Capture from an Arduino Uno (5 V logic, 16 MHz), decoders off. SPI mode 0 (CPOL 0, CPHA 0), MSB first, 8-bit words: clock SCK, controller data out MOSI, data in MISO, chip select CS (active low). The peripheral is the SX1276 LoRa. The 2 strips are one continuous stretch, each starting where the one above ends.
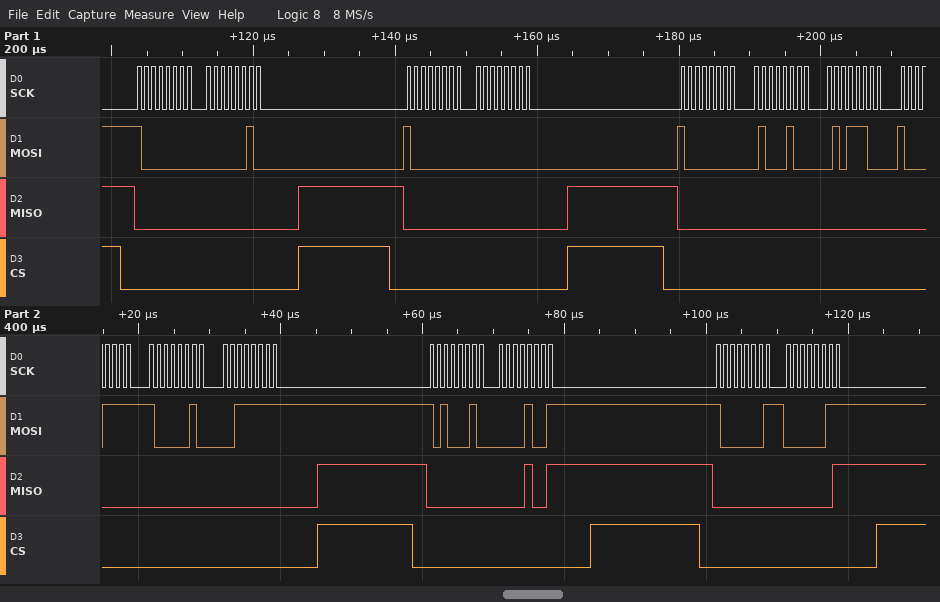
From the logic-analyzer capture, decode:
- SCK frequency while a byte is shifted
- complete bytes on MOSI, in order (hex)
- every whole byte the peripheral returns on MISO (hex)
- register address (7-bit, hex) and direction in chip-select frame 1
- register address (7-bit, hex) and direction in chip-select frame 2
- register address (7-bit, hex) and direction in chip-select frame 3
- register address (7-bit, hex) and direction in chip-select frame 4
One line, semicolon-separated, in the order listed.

1 MHz; 80 02 80 00 80 44 5C 8F 82 3F A2 09 81 03; 00 00 00 00 00 00 00 00 00 00 00 09 00 01; 0x00 write; 0x00 write; 0x00 write; 0x22 write
